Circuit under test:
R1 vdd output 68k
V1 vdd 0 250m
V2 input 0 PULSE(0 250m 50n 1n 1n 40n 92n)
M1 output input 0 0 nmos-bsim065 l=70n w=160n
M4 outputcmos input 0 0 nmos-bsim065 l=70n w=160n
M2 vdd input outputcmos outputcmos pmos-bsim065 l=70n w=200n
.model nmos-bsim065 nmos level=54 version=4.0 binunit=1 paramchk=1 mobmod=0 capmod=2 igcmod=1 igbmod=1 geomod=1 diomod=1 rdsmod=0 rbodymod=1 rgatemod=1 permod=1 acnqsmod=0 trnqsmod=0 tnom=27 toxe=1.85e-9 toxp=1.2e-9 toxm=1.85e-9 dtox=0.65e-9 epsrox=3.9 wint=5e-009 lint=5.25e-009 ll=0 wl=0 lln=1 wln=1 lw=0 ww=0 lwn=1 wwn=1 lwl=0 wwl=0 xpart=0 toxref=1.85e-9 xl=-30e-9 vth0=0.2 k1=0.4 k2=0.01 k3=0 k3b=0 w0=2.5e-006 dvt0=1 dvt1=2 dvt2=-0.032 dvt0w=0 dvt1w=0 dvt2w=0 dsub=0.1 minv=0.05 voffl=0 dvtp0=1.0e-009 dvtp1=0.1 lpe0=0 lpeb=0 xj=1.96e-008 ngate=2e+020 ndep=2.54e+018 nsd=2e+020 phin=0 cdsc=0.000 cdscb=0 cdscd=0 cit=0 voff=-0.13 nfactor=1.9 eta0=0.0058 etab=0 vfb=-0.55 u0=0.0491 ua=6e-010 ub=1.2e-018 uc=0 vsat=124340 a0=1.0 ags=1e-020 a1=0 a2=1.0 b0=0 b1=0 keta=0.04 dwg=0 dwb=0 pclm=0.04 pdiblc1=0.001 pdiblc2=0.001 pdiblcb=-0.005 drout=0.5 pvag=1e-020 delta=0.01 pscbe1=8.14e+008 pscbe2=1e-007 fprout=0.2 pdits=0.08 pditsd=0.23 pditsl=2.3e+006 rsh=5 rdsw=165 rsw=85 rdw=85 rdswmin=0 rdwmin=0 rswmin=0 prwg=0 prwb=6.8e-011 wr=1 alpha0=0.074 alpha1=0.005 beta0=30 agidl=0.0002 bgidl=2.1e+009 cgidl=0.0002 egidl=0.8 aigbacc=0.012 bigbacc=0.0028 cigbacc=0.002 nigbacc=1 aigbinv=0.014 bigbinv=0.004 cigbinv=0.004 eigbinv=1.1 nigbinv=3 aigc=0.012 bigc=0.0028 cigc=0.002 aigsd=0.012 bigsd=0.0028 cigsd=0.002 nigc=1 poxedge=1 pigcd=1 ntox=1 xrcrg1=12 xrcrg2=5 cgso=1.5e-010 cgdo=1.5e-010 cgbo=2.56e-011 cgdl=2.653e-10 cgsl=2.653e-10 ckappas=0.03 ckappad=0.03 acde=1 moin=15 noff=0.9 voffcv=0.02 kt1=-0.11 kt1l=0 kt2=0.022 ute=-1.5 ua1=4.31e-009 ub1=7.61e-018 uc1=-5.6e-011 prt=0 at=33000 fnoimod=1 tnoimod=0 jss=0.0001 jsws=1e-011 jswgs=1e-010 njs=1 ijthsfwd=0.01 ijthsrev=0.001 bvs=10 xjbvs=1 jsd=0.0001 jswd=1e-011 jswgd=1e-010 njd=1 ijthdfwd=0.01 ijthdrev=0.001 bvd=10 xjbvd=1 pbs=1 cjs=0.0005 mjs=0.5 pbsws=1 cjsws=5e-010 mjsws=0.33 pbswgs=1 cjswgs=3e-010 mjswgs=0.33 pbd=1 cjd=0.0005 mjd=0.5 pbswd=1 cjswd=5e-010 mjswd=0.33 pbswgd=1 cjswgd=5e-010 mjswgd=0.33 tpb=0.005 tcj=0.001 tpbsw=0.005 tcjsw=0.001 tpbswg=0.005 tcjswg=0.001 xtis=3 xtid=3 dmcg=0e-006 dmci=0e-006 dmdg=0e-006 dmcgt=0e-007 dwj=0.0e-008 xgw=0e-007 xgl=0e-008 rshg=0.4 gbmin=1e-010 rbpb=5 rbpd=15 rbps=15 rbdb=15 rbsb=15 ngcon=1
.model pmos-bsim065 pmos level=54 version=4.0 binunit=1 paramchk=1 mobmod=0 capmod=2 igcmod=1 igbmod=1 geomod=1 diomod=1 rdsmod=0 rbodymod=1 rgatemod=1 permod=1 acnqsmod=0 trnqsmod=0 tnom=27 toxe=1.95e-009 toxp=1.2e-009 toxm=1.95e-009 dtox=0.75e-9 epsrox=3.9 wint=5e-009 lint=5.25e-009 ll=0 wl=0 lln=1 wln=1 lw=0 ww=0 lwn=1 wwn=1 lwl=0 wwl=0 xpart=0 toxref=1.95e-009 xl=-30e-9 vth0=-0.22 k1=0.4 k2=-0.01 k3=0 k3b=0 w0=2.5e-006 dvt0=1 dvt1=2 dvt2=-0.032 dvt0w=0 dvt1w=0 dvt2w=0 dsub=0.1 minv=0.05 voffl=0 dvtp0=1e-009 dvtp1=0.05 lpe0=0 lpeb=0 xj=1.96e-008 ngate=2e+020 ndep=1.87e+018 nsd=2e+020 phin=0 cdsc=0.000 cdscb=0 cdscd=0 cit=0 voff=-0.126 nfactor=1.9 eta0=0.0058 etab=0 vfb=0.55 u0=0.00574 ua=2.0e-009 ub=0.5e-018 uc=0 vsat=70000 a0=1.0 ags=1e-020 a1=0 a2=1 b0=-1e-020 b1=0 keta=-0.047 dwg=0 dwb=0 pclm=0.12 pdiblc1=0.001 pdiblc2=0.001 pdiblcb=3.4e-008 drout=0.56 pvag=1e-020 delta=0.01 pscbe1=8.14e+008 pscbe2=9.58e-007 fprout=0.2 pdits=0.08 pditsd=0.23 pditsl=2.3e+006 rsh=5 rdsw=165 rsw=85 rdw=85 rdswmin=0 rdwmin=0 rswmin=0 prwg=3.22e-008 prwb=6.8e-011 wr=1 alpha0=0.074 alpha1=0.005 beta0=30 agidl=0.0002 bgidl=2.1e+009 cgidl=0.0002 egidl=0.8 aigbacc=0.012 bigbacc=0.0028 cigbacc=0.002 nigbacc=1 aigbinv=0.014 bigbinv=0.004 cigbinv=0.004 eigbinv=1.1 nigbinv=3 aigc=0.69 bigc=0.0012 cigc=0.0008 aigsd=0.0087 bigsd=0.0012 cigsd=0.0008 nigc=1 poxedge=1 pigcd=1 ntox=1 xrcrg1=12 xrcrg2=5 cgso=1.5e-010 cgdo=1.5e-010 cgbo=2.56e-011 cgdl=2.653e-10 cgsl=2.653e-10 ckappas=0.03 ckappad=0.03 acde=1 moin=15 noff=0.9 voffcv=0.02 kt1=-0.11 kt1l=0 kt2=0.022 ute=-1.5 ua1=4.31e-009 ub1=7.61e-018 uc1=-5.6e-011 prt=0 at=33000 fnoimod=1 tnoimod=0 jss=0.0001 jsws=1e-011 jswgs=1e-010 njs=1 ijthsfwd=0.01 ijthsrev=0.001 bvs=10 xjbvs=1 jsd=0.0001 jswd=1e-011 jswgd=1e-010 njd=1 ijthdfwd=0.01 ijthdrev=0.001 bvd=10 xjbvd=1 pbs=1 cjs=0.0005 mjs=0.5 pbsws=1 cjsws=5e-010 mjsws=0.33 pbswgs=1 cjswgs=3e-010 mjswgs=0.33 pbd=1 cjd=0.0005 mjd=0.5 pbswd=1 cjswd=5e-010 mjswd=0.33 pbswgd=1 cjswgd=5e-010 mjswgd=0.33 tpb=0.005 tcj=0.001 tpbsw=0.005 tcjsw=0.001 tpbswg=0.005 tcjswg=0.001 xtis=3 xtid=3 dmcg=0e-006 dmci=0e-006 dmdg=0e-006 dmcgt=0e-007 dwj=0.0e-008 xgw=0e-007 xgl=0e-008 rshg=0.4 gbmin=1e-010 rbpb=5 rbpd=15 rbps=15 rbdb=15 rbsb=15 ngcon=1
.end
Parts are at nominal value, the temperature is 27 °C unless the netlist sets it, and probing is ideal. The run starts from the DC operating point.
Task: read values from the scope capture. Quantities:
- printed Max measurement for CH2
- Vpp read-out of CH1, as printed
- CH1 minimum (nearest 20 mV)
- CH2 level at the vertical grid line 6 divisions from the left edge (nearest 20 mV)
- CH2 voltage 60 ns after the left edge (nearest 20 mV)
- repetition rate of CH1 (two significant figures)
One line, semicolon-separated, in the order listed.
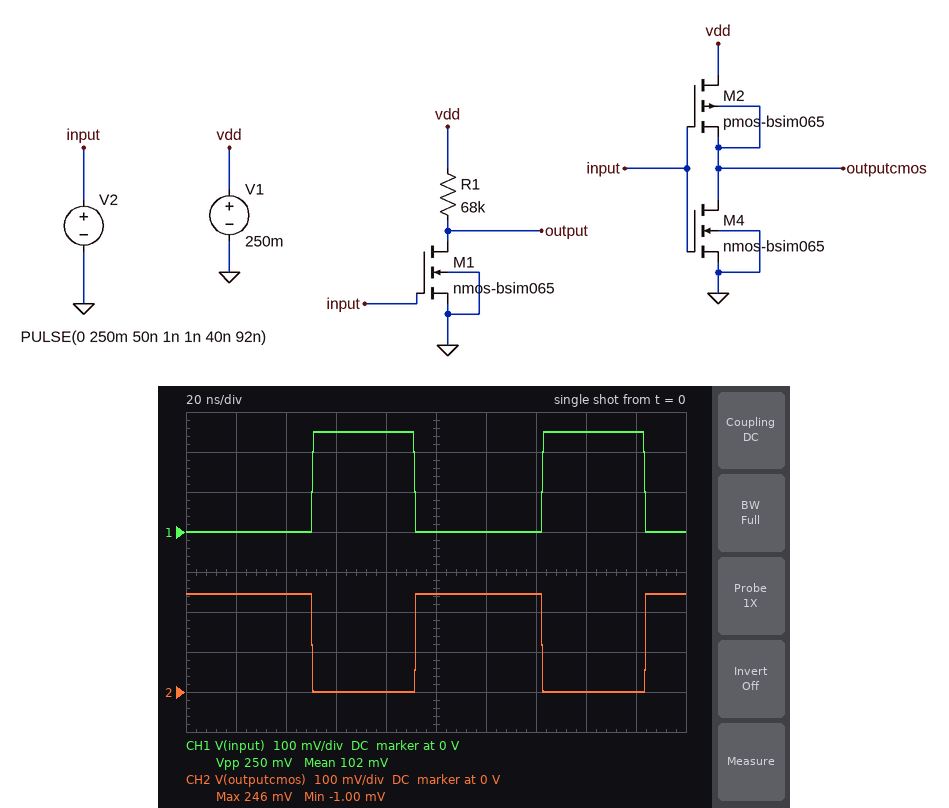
246 mV; 250 mV; 0 V; 240 mV; 0 V; 11 MHz
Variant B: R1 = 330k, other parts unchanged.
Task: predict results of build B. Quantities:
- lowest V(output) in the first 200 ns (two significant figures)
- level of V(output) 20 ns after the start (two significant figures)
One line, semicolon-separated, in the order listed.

3.9 mV; 220 mV
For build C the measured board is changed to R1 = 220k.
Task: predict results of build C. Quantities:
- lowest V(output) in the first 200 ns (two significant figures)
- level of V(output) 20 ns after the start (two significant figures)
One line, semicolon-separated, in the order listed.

6.0 mV; 230 mV
